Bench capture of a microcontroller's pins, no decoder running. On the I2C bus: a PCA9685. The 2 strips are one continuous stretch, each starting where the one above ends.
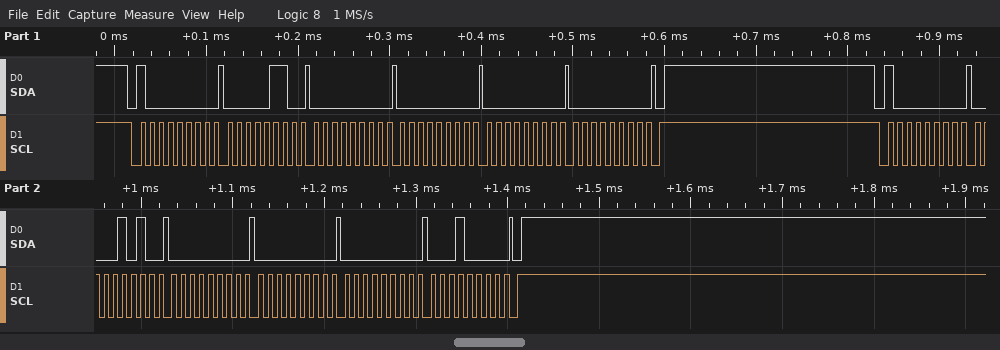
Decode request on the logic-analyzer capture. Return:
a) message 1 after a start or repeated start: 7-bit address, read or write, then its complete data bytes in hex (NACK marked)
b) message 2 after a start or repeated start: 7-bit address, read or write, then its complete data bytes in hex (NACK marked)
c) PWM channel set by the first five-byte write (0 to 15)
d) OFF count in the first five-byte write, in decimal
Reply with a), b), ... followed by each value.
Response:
a) 0x40 write: 06 00 00 00 00
b) 0x40 write: 0A 00 00 00 10
c) 0
d) 0
